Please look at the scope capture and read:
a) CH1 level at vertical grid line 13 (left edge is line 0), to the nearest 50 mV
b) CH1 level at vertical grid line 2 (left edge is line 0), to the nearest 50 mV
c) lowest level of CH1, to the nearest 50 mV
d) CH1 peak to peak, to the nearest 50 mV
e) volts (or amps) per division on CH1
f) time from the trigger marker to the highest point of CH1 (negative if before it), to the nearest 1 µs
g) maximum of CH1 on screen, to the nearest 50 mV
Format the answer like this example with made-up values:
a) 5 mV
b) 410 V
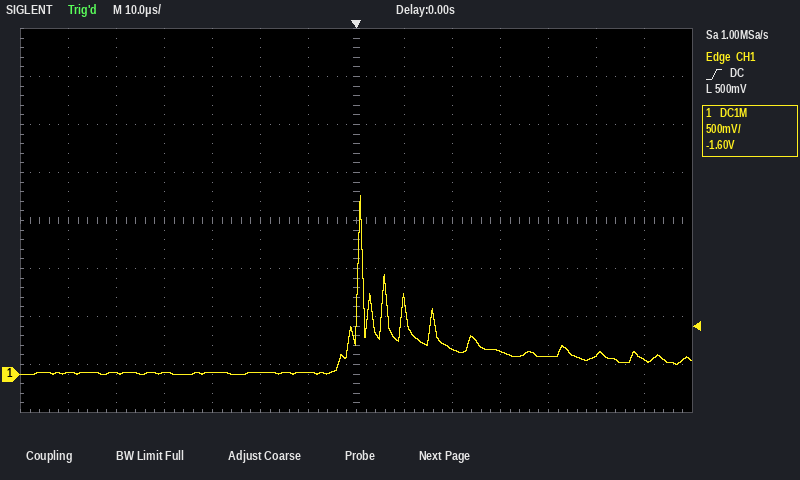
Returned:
a) 150 mV
b) 0 mV
c) 0 mV
d) 1.85 V
e) 500 mV
f) +1 µs
g) 1.85 V
